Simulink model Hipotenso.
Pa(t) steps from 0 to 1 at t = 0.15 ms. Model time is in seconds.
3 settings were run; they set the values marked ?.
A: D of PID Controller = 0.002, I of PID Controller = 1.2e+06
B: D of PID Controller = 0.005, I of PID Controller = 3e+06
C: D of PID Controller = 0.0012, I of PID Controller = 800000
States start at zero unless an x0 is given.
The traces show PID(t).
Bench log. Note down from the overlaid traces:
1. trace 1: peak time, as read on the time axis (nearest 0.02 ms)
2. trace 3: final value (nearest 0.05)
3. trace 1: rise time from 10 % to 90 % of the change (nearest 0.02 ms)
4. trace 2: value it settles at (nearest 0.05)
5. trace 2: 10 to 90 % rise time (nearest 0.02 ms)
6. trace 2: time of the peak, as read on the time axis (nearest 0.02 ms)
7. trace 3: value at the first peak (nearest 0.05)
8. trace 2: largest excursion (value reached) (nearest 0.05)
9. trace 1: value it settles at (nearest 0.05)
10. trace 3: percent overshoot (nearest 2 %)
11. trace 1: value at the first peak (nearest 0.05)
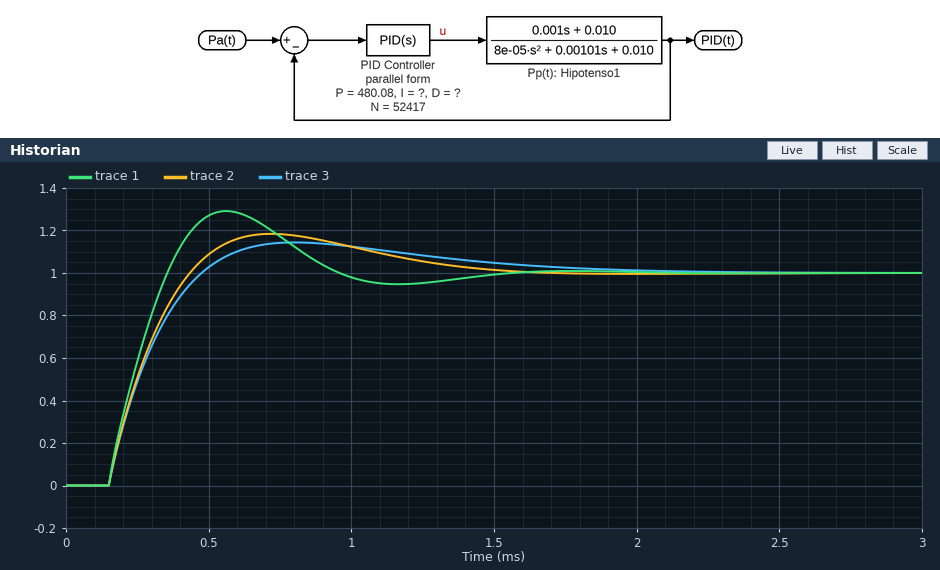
0.56 ms
1.00
0.16 ms
1.00
0.22 ms
0.72 ms
1.15
1.20
1.00
14 %
1.30
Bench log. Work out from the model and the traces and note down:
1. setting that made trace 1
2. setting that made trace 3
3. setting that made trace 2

B
C
A
